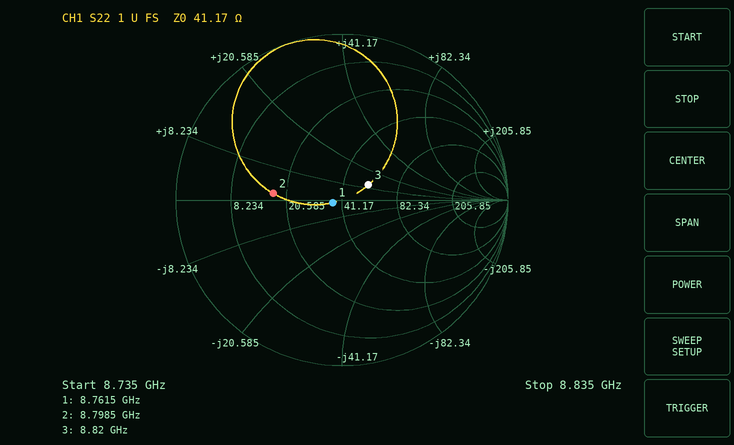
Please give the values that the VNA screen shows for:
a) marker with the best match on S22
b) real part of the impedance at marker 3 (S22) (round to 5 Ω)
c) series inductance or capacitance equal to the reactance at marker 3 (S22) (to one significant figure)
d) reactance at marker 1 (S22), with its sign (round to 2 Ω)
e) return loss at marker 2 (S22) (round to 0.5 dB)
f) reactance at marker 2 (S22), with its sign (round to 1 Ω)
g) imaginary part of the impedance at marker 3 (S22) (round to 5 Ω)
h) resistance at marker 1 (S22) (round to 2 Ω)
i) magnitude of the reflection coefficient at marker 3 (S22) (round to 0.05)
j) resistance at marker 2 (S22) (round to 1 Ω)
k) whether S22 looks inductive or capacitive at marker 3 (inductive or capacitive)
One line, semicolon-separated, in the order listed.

marker 1; 55 Ω; 200 pH; -2 Ω; 7.5 dB; +2 Ω; +10 Ω; 36 Ω; 0.20; 17 Ω; inductive
